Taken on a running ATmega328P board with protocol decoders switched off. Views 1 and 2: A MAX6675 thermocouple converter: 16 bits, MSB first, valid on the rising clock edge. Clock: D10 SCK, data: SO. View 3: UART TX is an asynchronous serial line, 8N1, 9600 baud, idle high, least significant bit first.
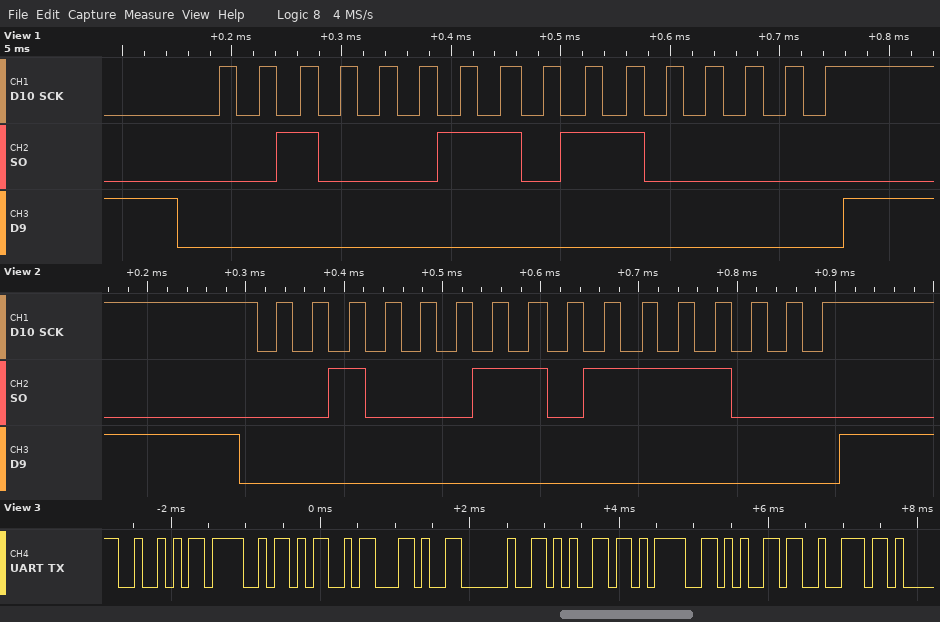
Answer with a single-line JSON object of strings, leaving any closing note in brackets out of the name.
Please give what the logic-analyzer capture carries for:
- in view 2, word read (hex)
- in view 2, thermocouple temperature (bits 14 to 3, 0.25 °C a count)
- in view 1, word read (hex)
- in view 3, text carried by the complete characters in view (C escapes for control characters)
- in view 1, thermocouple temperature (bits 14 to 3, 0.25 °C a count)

{"in view 2, word read": "0x2378", "in view 2, thermocouple temperature": "283.75 °C", "in view 1, word read": "0x2360", "in view 3, text carried by the complete characters in view": "\"ROM, e=er\"", "in view 1, thermocouple temperature": "283.00 °C"}
